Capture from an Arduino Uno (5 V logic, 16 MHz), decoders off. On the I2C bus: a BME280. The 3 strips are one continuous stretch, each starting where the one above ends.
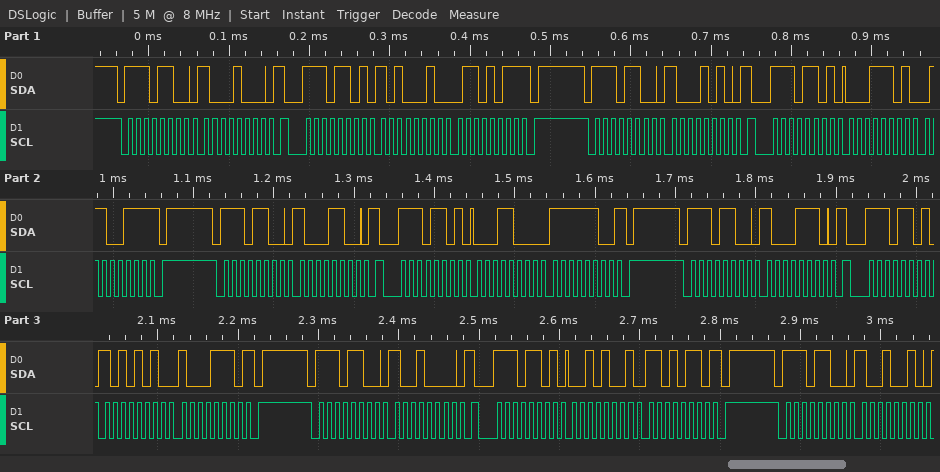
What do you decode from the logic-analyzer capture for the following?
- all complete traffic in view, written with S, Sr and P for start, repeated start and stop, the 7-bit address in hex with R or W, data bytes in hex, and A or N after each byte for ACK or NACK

S 76W A 88 A Sr 76R A A2 A 6B N P S 76W A 8A A Sr 76R A 1D A 67 N P S 76W A 8C A Sr 76R A 18 A FC N P S 76W A 8E A Sr 76R A AA A 8E N P S 76W A 90 A Sr 76R A 29 A D6 N P S 76W A 92 A
